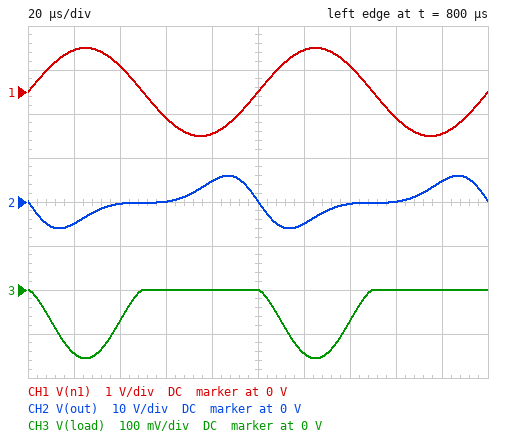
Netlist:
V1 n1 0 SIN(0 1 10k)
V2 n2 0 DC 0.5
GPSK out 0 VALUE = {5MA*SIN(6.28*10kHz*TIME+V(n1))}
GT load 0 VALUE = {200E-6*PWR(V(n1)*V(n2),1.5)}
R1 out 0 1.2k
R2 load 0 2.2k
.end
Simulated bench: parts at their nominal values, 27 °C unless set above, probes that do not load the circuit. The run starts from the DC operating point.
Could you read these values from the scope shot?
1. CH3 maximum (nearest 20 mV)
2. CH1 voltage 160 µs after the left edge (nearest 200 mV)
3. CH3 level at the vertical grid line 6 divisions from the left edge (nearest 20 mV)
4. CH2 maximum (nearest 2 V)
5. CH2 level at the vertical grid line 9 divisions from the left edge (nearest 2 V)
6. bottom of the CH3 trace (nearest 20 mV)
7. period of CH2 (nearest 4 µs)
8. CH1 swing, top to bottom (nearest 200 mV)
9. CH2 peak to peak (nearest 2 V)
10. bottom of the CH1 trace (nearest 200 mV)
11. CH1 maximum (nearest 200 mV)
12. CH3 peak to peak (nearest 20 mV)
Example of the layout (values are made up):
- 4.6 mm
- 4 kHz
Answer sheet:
- 0 V
- -600 mV
- -140 mV
- 6 V
- 4 V
- -160 mV
- 100 µs
- 2.0 V
- 12 V
- -1.0 V
- 1.0 V
- 160 mV
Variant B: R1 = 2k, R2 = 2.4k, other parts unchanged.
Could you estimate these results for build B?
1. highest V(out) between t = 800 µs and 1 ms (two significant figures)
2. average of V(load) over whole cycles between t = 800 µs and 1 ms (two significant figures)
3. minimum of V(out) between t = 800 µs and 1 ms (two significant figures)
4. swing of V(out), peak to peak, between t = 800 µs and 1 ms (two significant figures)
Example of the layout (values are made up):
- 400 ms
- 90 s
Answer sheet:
- 10 V
- -47 mV
- -10 V
- 20 V
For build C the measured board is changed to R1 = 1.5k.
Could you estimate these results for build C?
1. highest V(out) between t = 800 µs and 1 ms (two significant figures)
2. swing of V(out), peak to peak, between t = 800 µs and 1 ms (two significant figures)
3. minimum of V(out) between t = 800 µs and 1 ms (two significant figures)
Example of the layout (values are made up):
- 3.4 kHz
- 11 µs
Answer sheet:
- 7.5 V
- 15 V
- -7.5 V
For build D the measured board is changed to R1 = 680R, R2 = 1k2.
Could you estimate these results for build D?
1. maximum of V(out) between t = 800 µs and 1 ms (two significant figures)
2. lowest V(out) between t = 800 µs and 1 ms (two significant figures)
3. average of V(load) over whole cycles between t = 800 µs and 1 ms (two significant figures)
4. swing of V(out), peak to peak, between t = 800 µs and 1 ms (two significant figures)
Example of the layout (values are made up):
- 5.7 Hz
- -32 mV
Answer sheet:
- 3.4 V
- -3.4 V
- -24 mV
- 6.8 V
